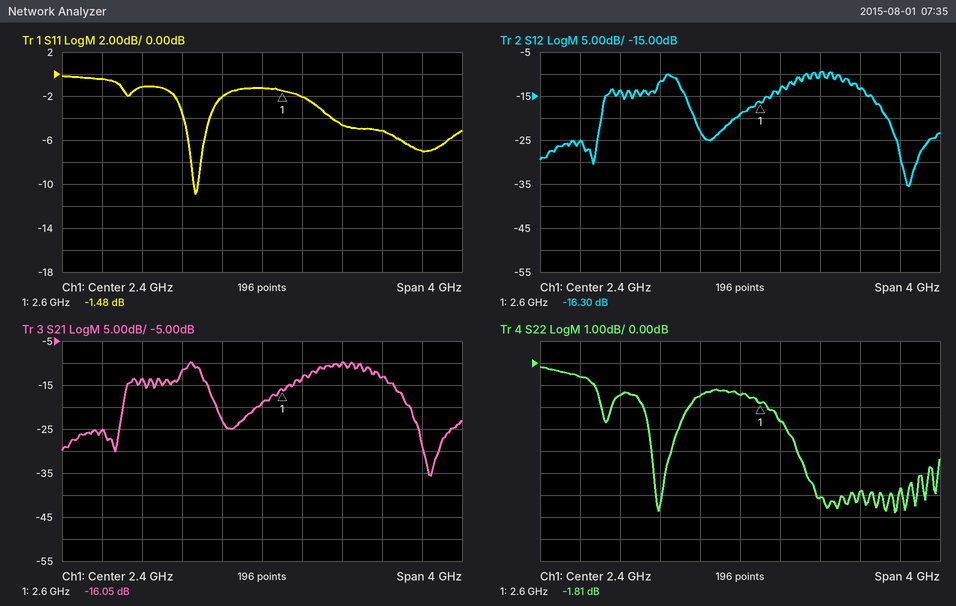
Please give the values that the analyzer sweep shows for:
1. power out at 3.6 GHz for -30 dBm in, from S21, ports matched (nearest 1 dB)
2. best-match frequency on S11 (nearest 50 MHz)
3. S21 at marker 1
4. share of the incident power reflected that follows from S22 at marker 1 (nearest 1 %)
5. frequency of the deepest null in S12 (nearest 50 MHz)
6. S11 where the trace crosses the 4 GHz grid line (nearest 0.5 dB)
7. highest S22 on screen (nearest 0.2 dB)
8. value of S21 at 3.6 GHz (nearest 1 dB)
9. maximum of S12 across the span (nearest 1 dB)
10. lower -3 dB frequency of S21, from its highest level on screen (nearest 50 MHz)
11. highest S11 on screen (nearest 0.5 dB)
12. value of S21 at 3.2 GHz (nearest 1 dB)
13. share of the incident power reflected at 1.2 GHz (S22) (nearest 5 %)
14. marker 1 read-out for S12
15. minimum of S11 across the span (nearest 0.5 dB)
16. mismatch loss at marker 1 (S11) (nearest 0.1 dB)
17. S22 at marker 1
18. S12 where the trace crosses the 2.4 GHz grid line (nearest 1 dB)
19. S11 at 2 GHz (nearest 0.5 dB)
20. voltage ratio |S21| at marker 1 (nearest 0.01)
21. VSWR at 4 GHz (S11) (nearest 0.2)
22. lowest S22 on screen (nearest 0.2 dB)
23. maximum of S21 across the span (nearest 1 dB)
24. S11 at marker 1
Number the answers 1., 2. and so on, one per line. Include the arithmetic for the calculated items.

1. -30 dBm + (-13 dB) = -43 dBm
2. 1.75 GHz
3. -16.05 dB
4. 10^(-1.81/10) ≈ 66 %
5. 4.10 GHz
6. -7.0 dB
7. -0.2 dB
8. -13 dB
9. -9 dB
10. 1.60 GHz
11. 0.0 dB
12. -10 dB
13. 10^(-1.4/10) ≈ 72.4 %, so 70 % to the nearest 5 %
14. -16.30 dB
15. -11.0 dB
16. −10 log10(1 − 10^(-1.48/10)) ≈ 5.4 dB
17. -1.81 dB
18. -19 dB
19. -2.0 dB
20. 10^(-16.05/20) ≈ 0.16
21. |Γ| = 10^(-7/20) = 0.4467; VSWR = (1 + 0.4467)/(1 − 0.4467) ≈ 2.6
22. -6.8 dB
23. -10 dB
24. -1.48 dB
